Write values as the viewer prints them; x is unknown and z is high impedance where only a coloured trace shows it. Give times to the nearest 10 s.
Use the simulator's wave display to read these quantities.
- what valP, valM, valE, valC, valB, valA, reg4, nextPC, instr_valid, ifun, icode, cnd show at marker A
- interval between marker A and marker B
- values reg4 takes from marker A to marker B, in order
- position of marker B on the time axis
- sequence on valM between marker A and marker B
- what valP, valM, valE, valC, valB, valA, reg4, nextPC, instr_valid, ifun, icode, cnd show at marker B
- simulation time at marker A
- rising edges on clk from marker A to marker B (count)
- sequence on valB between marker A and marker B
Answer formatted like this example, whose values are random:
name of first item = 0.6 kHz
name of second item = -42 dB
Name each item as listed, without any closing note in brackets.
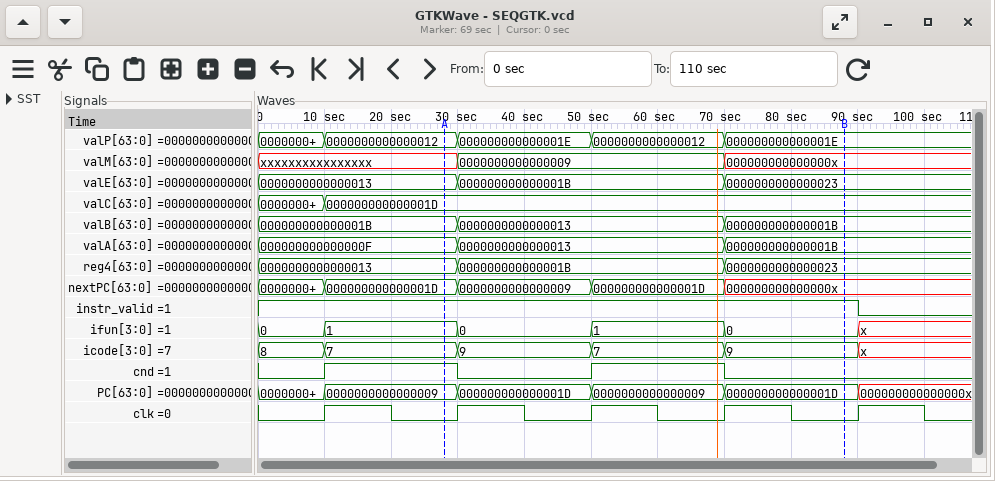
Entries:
what valP, valM, valE, valC, valB, valA, reg4, nextPC, instr_valid, ifun, icode, cnd show at marker A = valP=0000000000000012, valM=xxxxxxxxxxxxxxxx, valE=0000000000000013, valC=000000000000001D, valB=000000000000001B, valA=000000000000000F, reg4=0000000000000013, nextPC=000000000000001D, instr_valid=1, ifun=1, icode=7, cnd=1
interval between marker A and marker B = 60 s
values reg4 takes from marker A to marker B, in order = 0000000000000013, 000000000000001B, 0000000000000023
position of marker B on the time axis = 90 s
sequence on valM between marker A and marker B = xxxxxxxxxxxxxxxx, 0000000000000009, 000000000000000x
what valP, valM, valE, valC, valB, valA, reg4, nextPC, instr_valid, ifun, icode, cnd show at marker B = valP=000000000000001E, valM=000000000000000x, valE=0000000000000023, valC=000000000000001D, valB=000000000000001B, valA=000000000000001B, reg4=0000000000000023, nextPC=000000000000000x, instr_valid=1, ifun=0, icode=9, cnd=0
simulation time at marker A = 30 s
rising edges on clk from marker A to marker B = 3
sequence on valB between marker A and marker B = 000000000000001B, 0000000000000013, 000000000000001B
